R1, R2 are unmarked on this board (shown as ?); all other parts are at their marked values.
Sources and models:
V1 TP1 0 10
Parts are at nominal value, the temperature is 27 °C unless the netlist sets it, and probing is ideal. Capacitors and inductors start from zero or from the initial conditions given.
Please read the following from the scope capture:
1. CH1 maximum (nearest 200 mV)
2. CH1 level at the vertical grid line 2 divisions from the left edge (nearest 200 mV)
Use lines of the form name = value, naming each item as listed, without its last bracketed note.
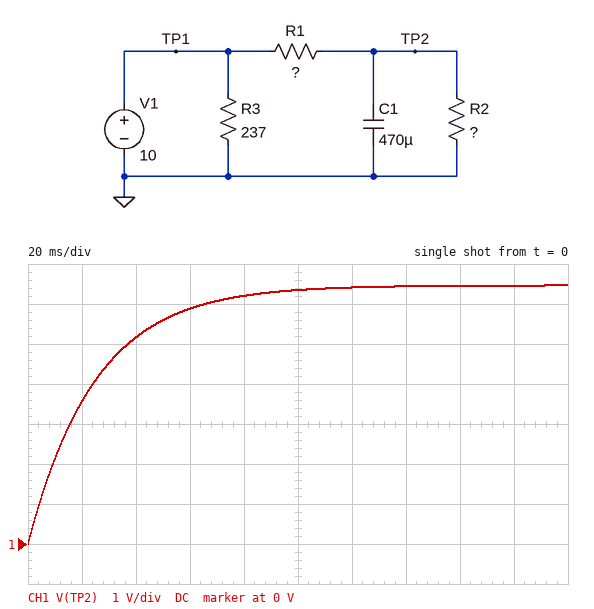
CH1 maximum = 6.4 V
CH1 level at the vertical grid line 2 divisions from the left edge = 5.2 V
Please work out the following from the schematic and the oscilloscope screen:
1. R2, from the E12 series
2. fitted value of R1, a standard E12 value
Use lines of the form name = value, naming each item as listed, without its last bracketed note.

R2, from the E12 series = 150 Ω
fitted value of R1, a standard E12 value = 82 Ω
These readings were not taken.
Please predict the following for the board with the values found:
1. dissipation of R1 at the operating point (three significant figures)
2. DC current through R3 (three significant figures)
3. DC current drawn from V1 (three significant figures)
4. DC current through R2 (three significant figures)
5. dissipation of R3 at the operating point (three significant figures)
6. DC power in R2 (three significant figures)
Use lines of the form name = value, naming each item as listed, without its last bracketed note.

dissipation of R1 at the operating point = 152 mW
DC current through R3 = 42.2 mA
DC current drawn from V1 = 85.3 mA
DC current through R2 = 43.1 mA
dissipation of R3 at the operating point = 422 mW
DC power in R2 = 279 mW
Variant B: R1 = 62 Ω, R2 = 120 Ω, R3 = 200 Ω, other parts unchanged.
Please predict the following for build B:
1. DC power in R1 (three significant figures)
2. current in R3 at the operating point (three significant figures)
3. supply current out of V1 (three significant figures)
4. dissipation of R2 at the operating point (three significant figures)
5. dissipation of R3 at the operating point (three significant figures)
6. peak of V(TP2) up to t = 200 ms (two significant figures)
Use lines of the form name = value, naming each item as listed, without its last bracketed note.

DC power in R1 = 187 mW
current in R3 at the operating point = 50.0 mA
supply current out of V1 = 105 mA
dissipation of R2 at the operating point = 362 mW
dissipation of R3 at the operating point = 500 mW
peak of V(TP2) up to t = 200 ms = 6.6 V
